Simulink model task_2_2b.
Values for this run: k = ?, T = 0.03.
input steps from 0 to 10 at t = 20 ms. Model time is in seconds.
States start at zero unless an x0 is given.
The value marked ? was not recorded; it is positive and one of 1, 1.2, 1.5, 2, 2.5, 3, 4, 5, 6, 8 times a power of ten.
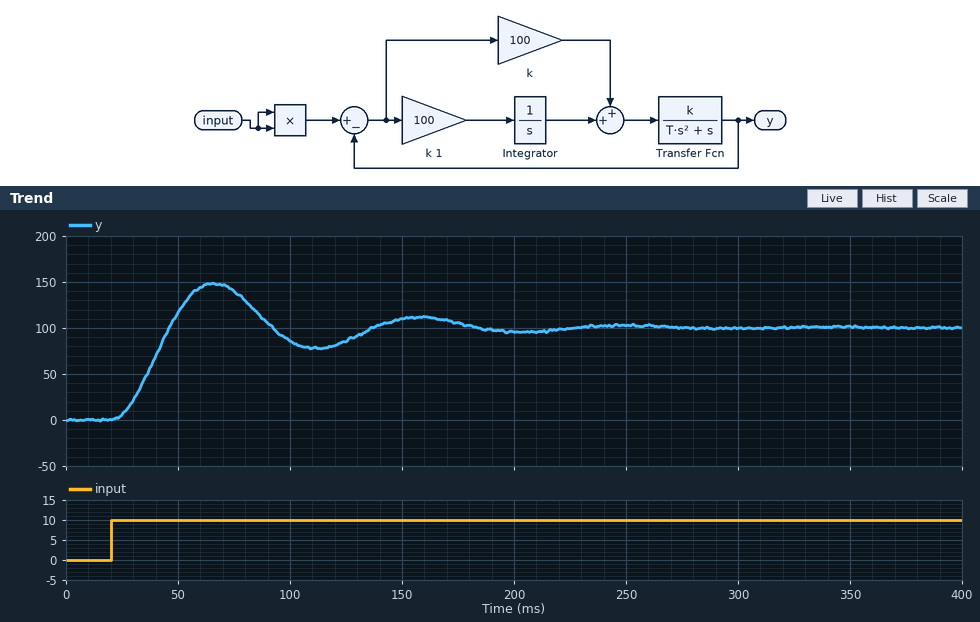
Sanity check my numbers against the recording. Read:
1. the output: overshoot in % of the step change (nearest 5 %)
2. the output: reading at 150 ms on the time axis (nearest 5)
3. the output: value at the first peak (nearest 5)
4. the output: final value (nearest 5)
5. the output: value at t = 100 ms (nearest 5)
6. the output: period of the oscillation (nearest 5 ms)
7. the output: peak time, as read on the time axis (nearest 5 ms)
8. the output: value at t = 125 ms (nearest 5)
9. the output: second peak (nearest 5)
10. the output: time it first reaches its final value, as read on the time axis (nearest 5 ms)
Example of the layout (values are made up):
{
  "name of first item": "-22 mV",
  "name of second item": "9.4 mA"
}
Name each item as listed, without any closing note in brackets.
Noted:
{
  "the output: overshoot in % of the step change": "50 %",
  "the output: reading at 150 ms on the time axis": "110",
  "the output: value at the first peak": "150",
  "the output: final value": "100",
  "the output: value at t = 100 ms": "85",
  "the output: period of the oscillation": "90 ms",
  "the output: peak time, as read on the time axis": "65 ms",
  "the output: value at t = 125 ms": "85",
  "the output: second peak": "110",
  "the output: time it first reaches its final value, as read on the time axis": "45 ms"
}
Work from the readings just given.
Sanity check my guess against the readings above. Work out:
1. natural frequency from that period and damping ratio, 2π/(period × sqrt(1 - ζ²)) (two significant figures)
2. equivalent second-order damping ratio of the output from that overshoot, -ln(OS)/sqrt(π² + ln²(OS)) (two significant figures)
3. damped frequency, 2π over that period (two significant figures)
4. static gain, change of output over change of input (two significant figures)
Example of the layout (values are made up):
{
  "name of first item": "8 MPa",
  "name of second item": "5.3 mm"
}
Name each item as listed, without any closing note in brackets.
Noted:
{
  "natural frequency from that period and damping ratio, 2π/(period × sqrt(1 - ζ²))": "0.072 rad/ms",
  "equivalent second-order damping ratio of the output from that overshoot, -ln(OS)/sqrt(π² + ln²(OS))": "0.22",
  "damped frequency, 2π over that period": "0.070 rad/ms",
  "static gain, change of output over change of input": "10"
}
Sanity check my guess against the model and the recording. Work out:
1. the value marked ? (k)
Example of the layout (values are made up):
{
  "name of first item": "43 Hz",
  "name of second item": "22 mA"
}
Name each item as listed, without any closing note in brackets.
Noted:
{
  "the value marked ?": "1.5"
}
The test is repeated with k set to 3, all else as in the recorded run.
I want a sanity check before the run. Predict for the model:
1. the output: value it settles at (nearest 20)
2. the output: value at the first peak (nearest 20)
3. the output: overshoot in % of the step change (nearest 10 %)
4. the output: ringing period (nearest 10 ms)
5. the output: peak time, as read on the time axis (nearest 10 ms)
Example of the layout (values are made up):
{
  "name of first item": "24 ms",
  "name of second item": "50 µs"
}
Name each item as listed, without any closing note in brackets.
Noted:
{
  "the output: value it settles at": "100",
  "the output: value at the first peak": "160",
  "the output: overshoot in % of the step change": "60 %",
  "the output: ringing period": "60 ms",
  "the output: peak time, as read on the time axis": "50 ms"
}
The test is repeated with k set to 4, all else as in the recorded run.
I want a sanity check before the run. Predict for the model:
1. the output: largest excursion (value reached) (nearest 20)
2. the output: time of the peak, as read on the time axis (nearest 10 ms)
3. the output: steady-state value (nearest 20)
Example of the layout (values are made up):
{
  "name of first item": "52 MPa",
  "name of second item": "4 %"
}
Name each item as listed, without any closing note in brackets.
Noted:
{
  "the output: largest excursion (value reached)": "160",
  "the output: time of the peak, as read on the time axis": "50 ms",
  "the output: steady-state value": "100"
}
